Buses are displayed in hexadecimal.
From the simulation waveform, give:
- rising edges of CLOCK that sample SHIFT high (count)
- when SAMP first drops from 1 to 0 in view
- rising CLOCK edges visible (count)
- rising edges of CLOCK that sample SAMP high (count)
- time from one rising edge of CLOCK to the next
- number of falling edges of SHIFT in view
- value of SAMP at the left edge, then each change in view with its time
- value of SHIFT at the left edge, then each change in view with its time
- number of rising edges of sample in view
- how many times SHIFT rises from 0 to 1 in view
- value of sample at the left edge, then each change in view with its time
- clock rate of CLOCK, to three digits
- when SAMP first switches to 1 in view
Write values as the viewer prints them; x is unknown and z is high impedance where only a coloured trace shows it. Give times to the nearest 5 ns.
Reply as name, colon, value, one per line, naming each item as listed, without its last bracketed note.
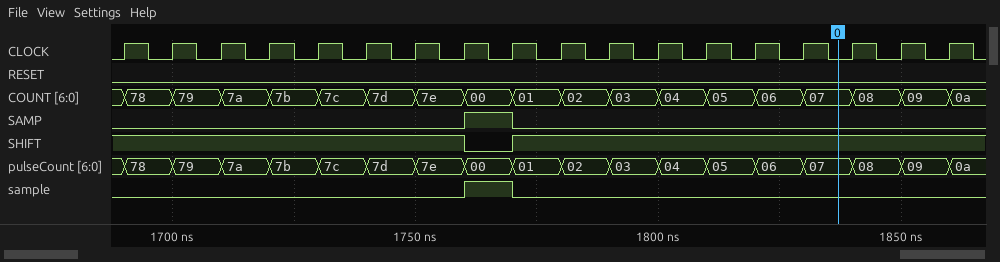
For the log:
rising edges of CLOCK that sample SHIFT high: 17
when SAMP first drops from 1 to 0 in view: 1770 ns
rising CLOCK edges visible: 18
rising edges of CLOCK that sample SAMP high: 1
time from one rising edge of CLOCK to the next: 10 ns
number of falling edges of SHIFT in view: 1
value of SAMP at the left edge, then each change in view with its time: 0, 1 at 1760 ns, 0 at 1770 ns
value of SHIFT at the left edge, then each change in view with its time: 1, 0 at 1760 ns, 1 at 1770 ns
number of rising edges of sample in view: 1
how many times SHIFT rises from 0 to 1 in view: 1
value of sample at the left edge, then each change in view with its time: 0, 1 at 1760 ns, 0 at 1770 ns
clock rate of CLOCK, to three digits: 100 MHz
when SAMP first switches to 1 in view: 1760 ns
